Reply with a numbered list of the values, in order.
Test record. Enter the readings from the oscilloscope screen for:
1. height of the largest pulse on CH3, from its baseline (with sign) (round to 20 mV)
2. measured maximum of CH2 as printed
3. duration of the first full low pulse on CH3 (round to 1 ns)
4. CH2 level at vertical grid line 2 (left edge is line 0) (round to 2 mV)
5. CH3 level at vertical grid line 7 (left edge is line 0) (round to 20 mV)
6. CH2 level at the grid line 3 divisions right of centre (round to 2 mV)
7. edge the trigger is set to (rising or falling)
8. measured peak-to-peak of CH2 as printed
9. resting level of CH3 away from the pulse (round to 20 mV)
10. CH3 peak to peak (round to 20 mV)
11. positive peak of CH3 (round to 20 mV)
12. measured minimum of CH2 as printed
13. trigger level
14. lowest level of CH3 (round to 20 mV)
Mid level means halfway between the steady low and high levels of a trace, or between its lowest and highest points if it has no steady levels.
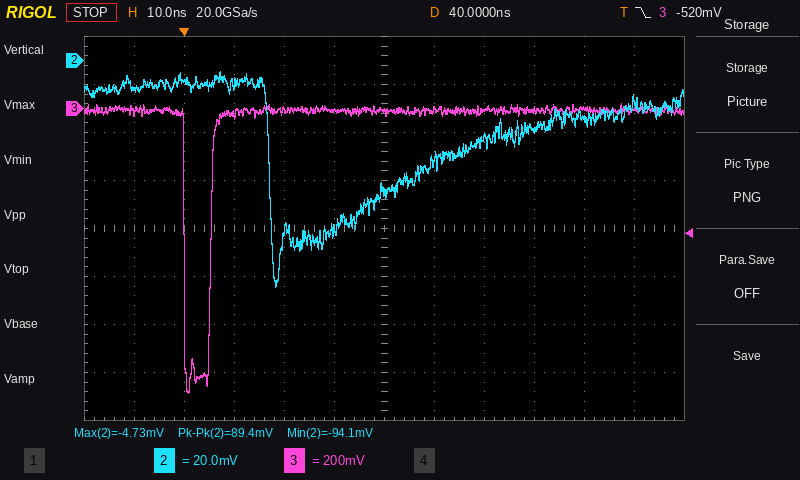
1. -1.18 V
2. -4.73 mV
3. 5 ns
4. -8 mV
5. 0 mV
6. -28 mV
7. falling
8. 89.4 mV
9. 0 mV
10. 1.20 V
11. 20 mV
12. -94.1 mV
13. -520 mV
14. -1.18 V
